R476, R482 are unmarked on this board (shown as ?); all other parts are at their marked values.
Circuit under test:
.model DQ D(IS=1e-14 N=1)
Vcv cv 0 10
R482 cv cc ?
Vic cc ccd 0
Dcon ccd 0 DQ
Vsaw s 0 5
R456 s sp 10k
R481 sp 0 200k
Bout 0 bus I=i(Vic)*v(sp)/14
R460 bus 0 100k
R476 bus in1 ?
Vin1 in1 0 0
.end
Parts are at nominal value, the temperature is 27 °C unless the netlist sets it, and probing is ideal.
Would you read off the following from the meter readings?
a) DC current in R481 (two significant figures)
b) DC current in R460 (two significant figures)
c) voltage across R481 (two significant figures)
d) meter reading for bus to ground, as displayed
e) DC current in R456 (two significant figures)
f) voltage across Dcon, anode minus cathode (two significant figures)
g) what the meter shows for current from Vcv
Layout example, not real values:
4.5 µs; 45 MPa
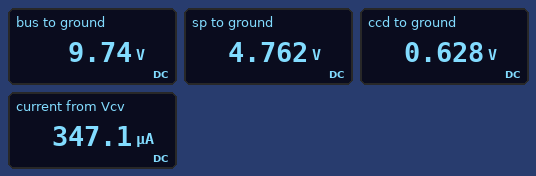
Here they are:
24 µA; 97 µA; 4.8 V; 9.74 V; 24 µA; 630 mV; 347.1 µA
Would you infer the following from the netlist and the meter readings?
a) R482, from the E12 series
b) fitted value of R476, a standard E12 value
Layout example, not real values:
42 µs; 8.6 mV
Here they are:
27 kΩ; 470 kΩ
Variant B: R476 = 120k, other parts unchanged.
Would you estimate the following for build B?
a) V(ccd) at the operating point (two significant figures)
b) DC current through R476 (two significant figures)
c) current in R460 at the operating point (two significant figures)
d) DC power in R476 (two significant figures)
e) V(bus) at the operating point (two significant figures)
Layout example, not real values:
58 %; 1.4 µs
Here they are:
630 mV; 54 µA; 64 µA; 350 µW; 6.4 V
